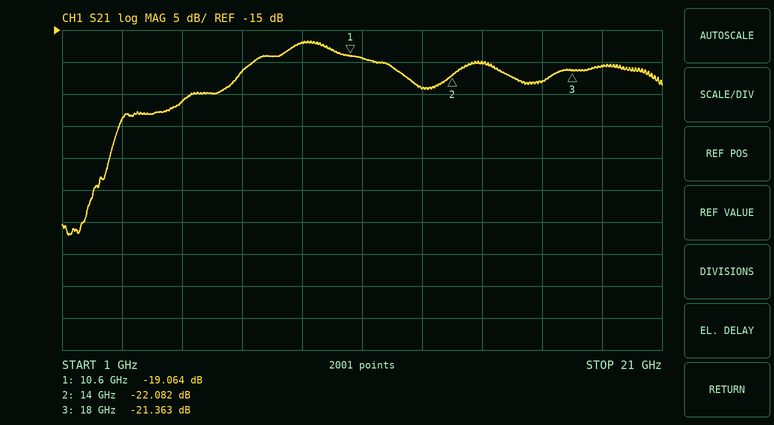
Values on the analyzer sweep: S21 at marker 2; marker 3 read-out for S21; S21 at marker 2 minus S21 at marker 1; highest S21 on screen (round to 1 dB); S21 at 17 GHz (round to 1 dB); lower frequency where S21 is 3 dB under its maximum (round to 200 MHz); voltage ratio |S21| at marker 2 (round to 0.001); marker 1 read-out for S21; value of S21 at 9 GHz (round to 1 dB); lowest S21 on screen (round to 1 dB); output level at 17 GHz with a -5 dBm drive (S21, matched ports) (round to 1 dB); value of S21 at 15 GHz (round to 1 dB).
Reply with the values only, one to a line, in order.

-22.082 dB
-21.363 dB
-3.018 dB
-17 dB
-23 dB
7.4 GHz
0.079
-19.064 dB
-17 dB
-47 dB
-28 dBm
-20 dB
